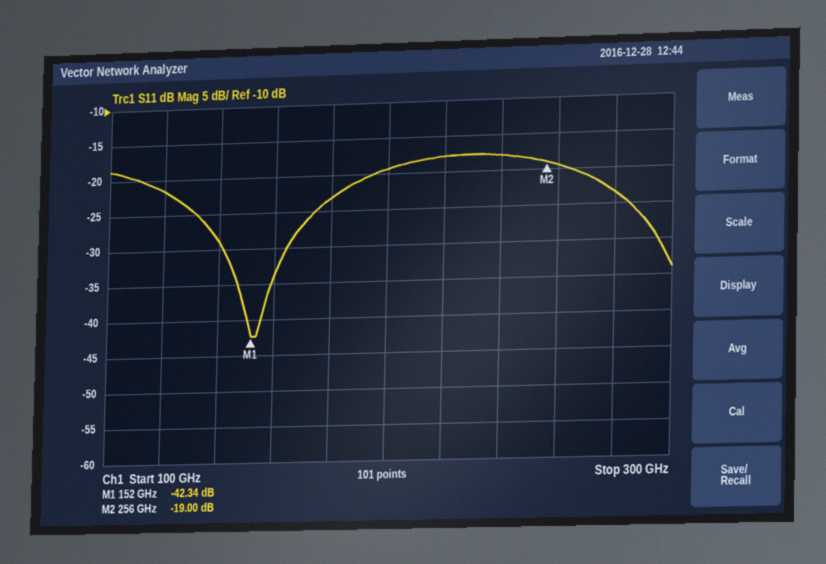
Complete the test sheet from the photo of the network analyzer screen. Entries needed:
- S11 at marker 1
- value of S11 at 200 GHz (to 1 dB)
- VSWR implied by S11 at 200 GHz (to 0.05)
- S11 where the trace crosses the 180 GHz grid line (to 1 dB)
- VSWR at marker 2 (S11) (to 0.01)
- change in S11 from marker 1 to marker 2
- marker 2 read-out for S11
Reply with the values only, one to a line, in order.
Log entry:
-42.34 dB
-19 dB
1.25
-23 dB
1.25
23.34 dB
-19.00 dB
